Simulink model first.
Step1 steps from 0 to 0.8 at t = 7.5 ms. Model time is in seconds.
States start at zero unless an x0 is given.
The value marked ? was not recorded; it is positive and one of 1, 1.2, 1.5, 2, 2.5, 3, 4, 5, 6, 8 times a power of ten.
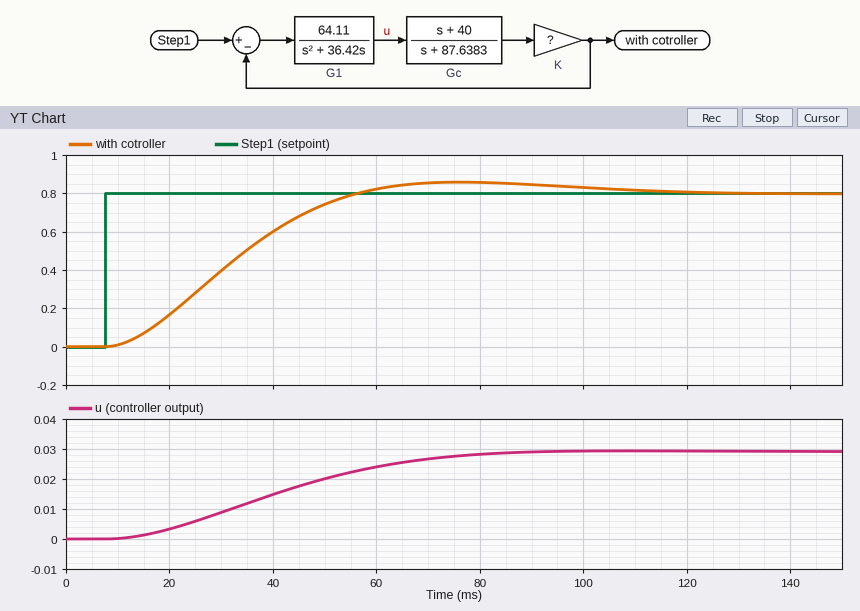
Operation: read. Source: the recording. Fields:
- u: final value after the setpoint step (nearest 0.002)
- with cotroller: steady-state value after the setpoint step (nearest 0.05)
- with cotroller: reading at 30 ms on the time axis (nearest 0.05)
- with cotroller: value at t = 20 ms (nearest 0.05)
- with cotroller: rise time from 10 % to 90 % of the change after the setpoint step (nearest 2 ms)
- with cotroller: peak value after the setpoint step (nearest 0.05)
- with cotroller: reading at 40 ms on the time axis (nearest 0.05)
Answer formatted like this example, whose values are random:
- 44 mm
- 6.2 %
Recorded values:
- 0.030
- 0.80
- 0.40
- 0.15
- 32 ms
- 0.85
- 0.60
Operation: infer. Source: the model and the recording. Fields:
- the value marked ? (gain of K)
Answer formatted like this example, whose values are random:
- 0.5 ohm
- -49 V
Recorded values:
- 60
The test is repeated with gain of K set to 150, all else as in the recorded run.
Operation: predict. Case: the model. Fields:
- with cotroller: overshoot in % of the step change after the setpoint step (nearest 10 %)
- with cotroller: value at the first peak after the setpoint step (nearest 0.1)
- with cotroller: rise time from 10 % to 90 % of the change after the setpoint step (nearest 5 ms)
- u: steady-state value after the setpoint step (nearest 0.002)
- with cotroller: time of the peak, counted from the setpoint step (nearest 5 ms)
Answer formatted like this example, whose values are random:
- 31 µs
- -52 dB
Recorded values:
- 20 %
- 1.0
- 15 ms
- 0.012
- 35 ms
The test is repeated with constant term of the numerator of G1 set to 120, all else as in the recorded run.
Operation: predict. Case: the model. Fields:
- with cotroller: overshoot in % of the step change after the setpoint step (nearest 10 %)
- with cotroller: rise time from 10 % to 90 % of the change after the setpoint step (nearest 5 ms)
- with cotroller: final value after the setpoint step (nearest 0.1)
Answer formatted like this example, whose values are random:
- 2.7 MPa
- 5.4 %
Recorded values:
- 20 %
- 20 ms
- 0.8
